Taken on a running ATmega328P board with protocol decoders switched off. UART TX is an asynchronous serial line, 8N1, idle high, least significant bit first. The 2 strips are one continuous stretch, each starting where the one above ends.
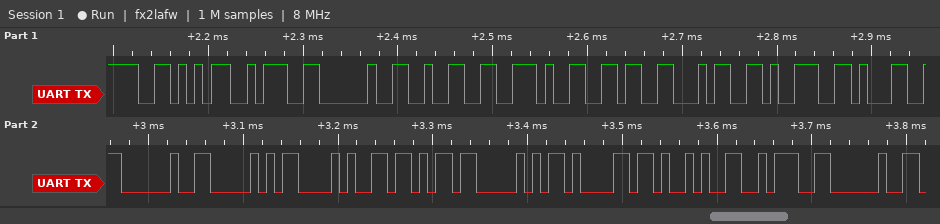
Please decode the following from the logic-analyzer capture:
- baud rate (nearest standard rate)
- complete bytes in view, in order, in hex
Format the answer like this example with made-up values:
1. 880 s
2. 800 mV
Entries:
1. 115200 baud
2. 56 3A 20 32 2E 36 34 39 31 20 50 28 6B 50 61 29 3A 20
